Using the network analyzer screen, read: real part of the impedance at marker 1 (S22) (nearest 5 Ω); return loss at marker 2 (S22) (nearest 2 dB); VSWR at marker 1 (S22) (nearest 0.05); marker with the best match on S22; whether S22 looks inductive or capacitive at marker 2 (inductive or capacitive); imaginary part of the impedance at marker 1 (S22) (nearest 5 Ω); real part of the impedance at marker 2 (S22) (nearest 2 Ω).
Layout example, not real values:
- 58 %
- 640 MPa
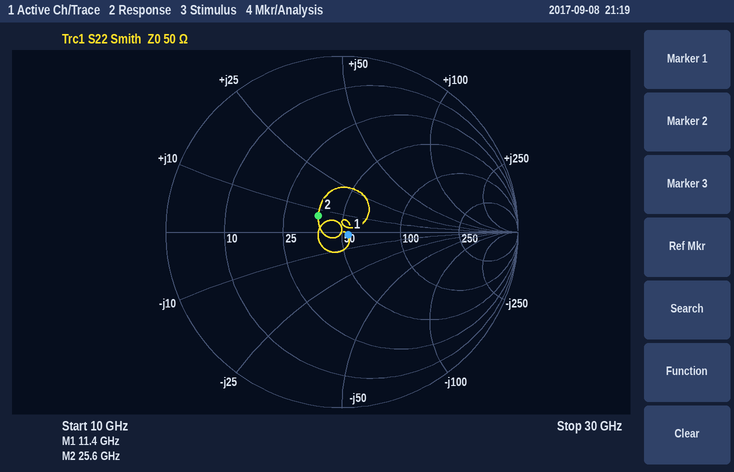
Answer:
- 55 Ω
- 16 dB
- 1.10
- marker 1
- inductive
- 0 Ω
- 38 Ω
